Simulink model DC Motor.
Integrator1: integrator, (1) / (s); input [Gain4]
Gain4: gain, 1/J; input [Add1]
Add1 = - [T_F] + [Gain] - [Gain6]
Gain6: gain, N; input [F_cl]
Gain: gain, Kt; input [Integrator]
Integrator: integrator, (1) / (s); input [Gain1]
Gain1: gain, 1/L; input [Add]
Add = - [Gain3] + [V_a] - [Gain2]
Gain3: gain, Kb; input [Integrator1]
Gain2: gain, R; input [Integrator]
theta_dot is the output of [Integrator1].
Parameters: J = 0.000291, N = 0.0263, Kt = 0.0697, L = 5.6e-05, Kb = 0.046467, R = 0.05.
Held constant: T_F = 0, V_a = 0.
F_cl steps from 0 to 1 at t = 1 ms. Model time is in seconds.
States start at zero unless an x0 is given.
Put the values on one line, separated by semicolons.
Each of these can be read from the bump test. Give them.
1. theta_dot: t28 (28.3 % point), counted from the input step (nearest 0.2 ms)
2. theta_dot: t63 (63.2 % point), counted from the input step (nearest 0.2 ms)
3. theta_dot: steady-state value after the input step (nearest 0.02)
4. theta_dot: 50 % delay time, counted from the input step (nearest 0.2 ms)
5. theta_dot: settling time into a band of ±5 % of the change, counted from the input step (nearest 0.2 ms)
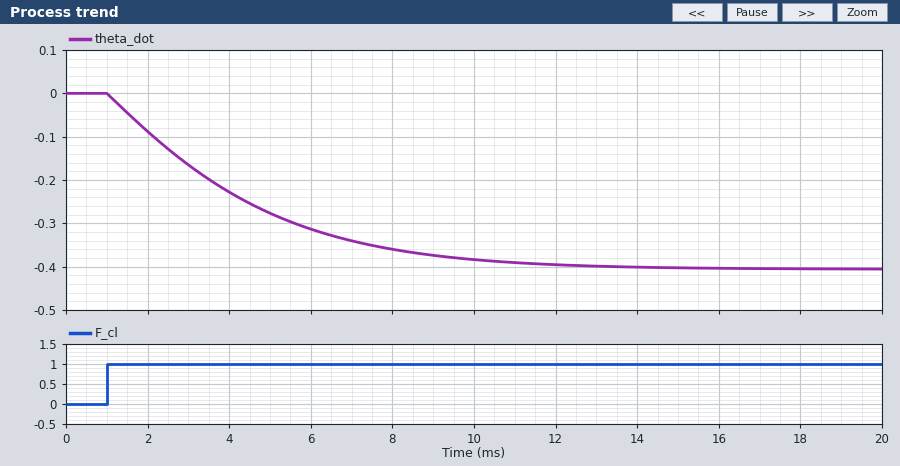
1.4 ms; 3.6 ms; -0.40; 2.6 ms; 9.2 ms
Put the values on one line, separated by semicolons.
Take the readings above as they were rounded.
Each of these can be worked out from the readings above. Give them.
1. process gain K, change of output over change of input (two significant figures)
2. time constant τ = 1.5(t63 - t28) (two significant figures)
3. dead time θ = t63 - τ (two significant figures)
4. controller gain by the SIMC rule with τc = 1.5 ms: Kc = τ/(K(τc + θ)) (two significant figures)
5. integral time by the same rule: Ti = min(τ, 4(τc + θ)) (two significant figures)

-0.40; 3.3 ms; 0.30 ms; -4.6; 3.3 ms
